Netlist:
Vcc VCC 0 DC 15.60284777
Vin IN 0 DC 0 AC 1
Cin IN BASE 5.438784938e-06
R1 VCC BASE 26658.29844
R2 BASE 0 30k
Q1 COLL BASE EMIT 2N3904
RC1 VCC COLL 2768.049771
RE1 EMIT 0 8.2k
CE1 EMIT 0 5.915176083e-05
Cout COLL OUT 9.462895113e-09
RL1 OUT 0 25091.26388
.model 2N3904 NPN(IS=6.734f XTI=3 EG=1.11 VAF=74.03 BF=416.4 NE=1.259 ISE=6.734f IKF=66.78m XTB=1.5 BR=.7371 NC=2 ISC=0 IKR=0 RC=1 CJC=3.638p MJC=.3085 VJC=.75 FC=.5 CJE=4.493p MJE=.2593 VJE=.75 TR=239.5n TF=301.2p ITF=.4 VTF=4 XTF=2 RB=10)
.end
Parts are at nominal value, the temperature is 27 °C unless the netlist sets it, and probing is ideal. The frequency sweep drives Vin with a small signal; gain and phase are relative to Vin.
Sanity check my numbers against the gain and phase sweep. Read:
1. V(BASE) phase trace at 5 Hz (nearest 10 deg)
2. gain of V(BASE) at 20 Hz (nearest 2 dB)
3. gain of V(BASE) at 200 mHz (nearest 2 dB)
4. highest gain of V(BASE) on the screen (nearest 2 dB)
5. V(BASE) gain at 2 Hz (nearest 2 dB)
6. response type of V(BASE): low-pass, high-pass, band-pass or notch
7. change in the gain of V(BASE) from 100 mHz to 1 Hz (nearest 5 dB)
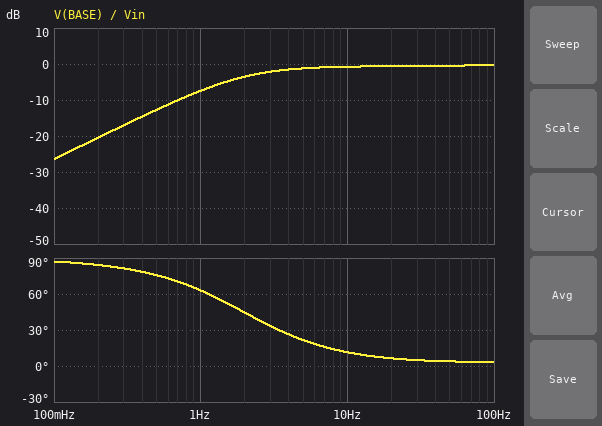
20 deg
0 dB
-20 dB
0 dB
-4 dB
high-pass
20 dB
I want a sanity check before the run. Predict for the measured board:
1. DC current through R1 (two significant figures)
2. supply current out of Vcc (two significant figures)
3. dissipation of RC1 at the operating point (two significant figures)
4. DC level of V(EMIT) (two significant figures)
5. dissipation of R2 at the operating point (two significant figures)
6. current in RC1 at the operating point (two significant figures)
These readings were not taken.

280 µA
1.2 mA
2.3 mW
7.5 V
2.2 mW
910 µA
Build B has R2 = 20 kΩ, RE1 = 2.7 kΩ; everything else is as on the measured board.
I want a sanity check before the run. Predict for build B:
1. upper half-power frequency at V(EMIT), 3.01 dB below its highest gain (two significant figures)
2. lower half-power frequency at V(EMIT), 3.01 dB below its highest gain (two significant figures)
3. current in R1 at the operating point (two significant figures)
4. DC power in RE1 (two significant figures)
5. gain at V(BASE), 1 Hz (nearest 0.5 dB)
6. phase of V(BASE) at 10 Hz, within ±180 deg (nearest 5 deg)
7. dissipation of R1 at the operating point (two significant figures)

220 Hz
2.4 Hz
340 µA
13 mW
-9.0 dB
15 deg
3.1 mW
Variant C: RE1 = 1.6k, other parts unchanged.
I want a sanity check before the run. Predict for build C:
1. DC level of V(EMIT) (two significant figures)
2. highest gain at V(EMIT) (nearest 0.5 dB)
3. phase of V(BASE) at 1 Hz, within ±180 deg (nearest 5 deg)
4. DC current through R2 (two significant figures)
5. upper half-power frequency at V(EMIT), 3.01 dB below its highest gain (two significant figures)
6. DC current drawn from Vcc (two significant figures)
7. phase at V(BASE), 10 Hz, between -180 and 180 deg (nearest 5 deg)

5.8 V
-21.0 dB
70 deg
220 µA
1.4 kHz
3.8 mA
20 deg
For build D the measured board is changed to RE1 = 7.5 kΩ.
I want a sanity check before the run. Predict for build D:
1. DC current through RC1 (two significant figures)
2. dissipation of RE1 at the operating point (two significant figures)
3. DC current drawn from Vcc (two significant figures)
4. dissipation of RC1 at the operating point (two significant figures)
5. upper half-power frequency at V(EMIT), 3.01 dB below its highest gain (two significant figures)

990 µA
7.5 mW
1.3 mA
2.7 mW
110 Hz
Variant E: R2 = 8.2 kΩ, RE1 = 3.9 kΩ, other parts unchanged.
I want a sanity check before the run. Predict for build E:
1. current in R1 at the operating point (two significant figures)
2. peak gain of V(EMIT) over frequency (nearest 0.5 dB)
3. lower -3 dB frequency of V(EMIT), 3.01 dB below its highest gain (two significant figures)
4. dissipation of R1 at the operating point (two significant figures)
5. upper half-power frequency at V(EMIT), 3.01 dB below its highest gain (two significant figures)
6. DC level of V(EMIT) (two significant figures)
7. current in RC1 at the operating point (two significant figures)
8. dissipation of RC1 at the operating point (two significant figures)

450 µA
-1.0 dB
4.0 Hz
5.4 mW
91 Hz
3.0 V
760 µA
1.6 mW
